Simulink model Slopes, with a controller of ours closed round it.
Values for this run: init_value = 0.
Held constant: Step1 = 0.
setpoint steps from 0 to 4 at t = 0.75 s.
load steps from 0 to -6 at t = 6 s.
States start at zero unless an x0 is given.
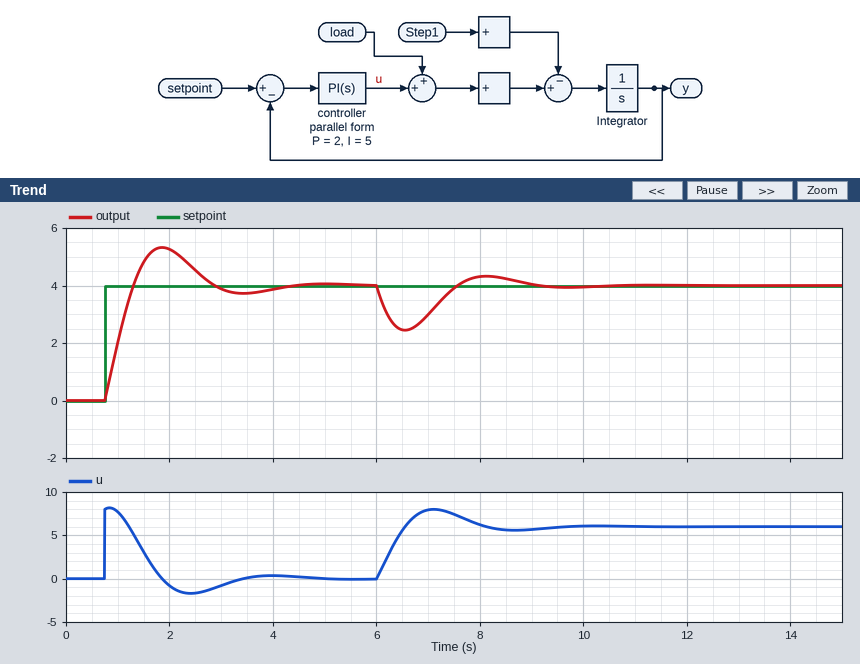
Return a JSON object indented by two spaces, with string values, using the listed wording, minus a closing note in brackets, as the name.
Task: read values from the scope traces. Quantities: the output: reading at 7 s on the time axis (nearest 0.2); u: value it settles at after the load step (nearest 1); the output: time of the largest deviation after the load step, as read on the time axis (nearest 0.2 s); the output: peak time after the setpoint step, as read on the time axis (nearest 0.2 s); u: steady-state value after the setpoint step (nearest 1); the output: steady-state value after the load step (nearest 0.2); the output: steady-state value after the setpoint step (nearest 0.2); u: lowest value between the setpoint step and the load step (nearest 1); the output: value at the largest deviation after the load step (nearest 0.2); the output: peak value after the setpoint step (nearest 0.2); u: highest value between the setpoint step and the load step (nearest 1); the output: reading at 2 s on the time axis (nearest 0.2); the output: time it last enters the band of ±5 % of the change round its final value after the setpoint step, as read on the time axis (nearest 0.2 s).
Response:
{
  "the output: reading at 7 s on the time axis": "3.0",
  "u: value it settles at after the load step": "6",
  "the output: time of the largest deviation after the load step, as read on the time axis": "6.6 s",
  "the output: peak time after the setpoint step, as read on the time axis": "1.8 s",
  "u: steady-state value after the setpoint step": "0",
  "the output: steady-state value after the load step": "4.0",
  "the output: steady-state value after the setpoint step": "4.0",
  "u: lowest value between the setpoint step and the load step": "-2",
  "the output: value at the largest deviation after the load step": "2.4",
  "the output: peak value after the setpoint step": "5.4",
  "u: highest value between the setpoint step and the load step": "8",
  "the output: reading at 2 s on the time axis": "5.2",
  "the output: time it last enters the band of ±5 % of the change round its final value after the setpoint step, as read on the time axis": "3.8 s"
}
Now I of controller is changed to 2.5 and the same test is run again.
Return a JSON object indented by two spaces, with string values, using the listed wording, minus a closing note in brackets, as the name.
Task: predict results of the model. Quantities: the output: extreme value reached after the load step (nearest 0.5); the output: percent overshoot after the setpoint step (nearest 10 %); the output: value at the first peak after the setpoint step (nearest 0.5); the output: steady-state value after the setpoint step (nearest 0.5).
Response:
{
  "the output: extreme value reached after the load step": "2.0",
  "the output: percent overshoot after the setpoint step": "20 %",
  "the output: value at the first peak after the setpoint step": "5.0",
  "the output: steady-state value after the setpoint step": "4.0"
}
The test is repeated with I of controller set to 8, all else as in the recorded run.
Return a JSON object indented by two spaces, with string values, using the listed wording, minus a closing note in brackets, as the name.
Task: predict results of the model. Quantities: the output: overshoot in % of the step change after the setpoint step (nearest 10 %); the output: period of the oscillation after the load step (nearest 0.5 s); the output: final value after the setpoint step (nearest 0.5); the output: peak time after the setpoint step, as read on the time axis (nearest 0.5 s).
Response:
{
  "the output: overshoot in % of the step change after the setpoint step": "40 %",
  "the output: period of the oscillation after the load step": "2.5 s",
  "the output: final value after the setpoint step": "4.0",
  "the output: peak time after the setpoint step, as read on the time axis": "1.5 s"
}
